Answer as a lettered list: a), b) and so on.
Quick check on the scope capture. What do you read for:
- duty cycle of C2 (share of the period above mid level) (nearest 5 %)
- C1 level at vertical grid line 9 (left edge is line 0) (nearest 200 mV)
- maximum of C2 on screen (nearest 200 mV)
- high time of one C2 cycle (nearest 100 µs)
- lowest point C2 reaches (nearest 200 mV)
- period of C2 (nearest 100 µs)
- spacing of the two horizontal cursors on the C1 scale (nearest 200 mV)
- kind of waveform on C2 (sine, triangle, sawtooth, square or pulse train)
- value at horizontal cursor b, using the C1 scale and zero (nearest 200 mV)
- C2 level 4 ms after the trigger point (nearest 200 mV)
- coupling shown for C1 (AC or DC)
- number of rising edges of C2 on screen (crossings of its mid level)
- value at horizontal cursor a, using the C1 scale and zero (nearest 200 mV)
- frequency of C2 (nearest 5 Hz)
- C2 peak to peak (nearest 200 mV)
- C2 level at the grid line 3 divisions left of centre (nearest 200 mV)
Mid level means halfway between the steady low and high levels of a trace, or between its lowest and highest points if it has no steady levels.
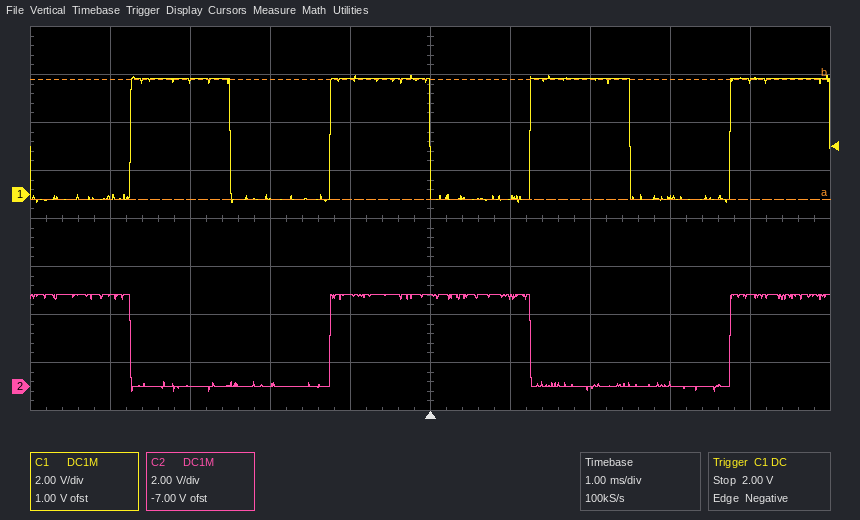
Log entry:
a) 50 %
b) 4.8 V
c) 3.8 V
d) 2.5 ms
e) -200 mV
f) 5.0 ms
g) 5.0 V
h) square
i) 4.8 V
j) 3.8 V
k) DC
l) 2
m) -200 mV
n) 200 Hz
o) 4.0 V
p) 0.0 V
